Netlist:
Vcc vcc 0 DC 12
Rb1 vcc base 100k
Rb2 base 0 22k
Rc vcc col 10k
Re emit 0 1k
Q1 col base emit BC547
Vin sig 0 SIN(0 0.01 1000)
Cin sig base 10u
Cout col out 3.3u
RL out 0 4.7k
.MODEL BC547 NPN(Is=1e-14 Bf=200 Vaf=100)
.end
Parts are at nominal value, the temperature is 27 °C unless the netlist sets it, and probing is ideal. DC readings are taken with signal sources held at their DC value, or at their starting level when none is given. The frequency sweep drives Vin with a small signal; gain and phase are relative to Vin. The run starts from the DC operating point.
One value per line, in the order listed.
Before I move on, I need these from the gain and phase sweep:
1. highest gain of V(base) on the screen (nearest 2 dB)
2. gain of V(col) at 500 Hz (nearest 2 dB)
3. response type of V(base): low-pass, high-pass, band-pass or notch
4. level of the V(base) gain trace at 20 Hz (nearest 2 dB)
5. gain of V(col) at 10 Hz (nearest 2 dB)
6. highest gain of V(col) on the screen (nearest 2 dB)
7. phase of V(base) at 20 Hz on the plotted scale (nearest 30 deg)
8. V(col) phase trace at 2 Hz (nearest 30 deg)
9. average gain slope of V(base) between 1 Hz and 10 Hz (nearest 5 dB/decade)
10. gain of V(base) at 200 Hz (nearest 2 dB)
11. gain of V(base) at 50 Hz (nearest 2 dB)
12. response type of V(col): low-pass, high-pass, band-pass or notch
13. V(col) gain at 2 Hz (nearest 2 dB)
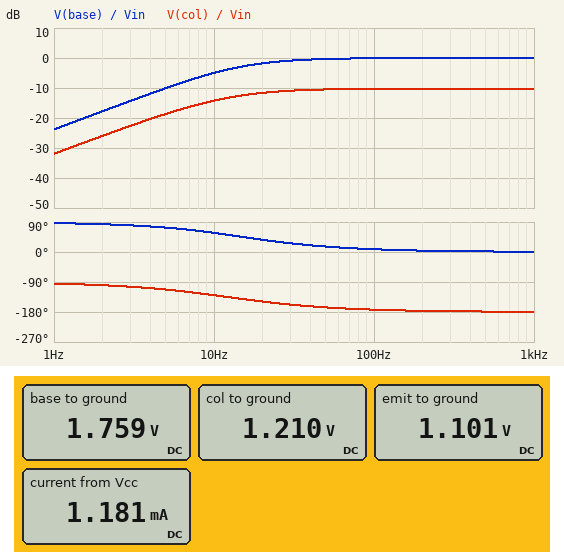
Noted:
0 dB
-10 dB
high-pass
-2 dB
-14 dB
-10 dB
30 deg
-90 deg
20 dB/decade
0 dB
0 dB
high-pass
-26 dB
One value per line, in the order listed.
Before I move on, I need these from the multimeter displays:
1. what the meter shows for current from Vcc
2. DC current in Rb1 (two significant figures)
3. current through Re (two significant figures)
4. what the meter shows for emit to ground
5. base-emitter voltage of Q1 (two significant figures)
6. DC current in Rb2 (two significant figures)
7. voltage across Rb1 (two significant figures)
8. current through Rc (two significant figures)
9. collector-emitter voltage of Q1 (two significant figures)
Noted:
1.181 mA
100 µA
1.1 mA
1.101 V
660 mV
80 µA
10 V
1.1 mA
110 mV
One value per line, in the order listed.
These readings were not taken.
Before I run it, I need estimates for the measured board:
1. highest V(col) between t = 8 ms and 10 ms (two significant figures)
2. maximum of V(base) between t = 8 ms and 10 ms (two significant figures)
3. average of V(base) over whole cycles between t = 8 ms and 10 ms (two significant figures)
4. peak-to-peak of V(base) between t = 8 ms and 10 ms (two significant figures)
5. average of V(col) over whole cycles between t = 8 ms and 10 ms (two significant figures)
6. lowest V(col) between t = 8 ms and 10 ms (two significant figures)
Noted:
1.2 V
1.8 V
1.8 V
20 mV
1.2 V
1.2 V
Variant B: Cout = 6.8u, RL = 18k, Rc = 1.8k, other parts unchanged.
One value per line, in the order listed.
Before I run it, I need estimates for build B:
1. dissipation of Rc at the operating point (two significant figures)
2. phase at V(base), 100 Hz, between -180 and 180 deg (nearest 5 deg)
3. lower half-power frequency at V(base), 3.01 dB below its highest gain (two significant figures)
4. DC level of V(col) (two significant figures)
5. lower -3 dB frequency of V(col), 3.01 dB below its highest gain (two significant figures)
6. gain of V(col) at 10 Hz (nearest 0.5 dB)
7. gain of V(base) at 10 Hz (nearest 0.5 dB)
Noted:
3.4 mW
0 deg
960 mHz
9.5 V
850 mHz
4.0 dB
0 dB
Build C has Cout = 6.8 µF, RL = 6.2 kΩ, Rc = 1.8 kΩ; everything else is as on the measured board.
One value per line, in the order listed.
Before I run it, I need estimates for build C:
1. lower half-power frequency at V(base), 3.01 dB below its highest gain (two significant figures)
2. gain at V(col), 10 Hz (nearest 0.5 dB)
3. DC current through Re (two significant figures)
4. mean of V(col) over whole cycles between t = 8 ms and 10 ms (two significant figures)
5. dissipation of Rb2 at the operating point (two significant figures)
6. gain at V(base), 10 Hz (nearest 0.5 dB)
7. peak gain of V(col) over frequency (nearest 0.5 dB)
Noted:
960 mHz
3.0 dB
1.4 mA
9.5 V
190 µW
0 dB
3.5 dB
